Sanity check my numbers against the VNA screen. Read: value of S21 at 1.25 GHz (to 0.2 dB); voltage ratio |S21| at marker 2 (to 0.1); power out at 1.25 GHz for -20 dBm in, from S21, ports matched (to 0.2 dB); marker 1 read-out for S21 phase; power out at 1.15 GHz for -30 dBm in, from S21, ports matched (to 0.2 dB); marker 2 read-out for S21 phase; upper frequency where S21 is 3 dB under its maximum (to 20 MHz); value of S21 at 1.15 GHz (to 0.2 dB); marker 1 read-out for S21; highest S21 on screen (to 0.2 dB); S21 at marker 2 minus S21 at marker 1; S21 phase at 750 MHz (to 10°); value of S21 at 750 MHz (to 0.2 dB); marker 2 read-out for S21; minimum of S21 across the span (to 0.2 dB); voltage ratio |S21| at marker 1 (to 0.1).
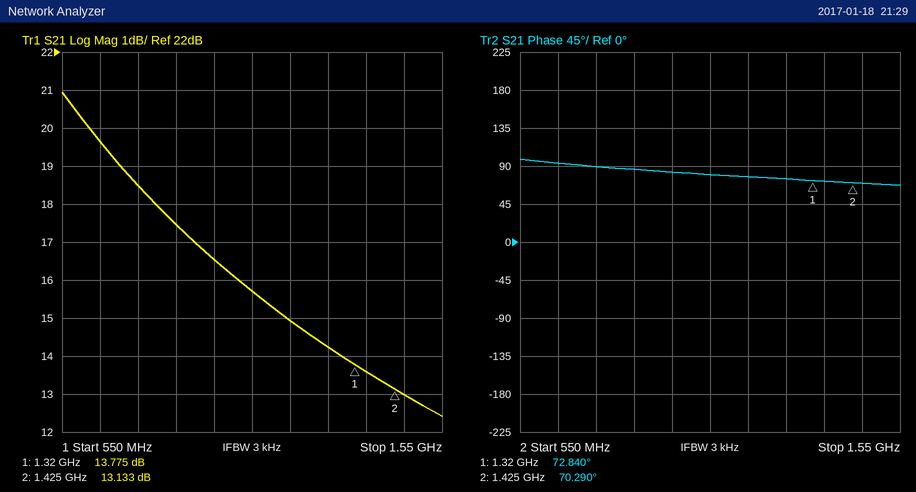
14.2 dB
4.5
-5.8 dBm
72.840°
-15.0 dBm
70.290°
800 MHz
15.0 dB
13.775 dB
21.0 dB
-0.642 dB
90°
18.4 dB
13.133 dB
12.4 dB
4.9
